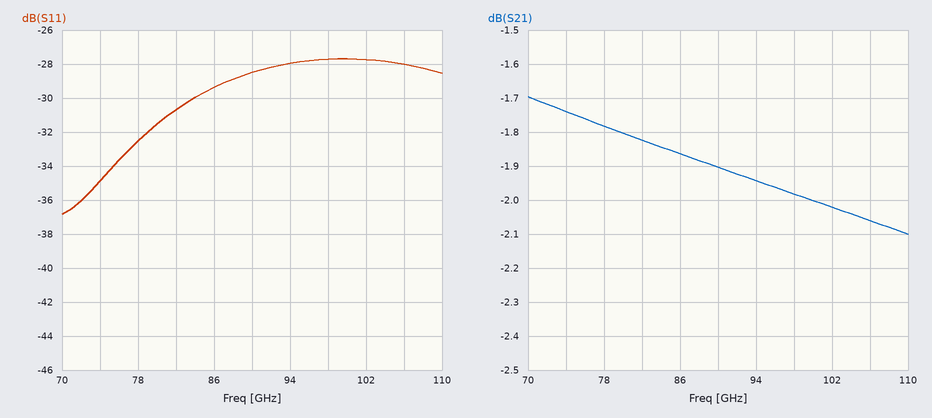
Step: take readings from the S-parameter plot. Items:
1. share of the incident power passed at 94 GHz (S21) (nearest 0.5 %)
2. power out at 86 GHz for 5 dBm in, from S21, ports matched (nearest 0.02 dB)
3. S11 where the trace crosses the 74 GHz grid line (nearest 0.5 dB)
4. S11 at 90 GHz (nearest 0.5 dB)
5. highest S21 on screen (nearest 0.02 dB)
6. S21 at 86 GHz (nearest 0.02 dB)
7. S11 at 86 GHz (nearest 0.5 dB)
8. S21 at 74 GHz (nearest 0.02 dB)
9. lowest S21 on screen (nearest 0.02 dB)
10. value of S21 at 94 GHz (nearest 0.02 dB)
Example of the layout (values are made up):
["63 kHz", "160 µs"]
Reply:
["64.0 %", "3.14 dBm", "-35.0 dB", "-28.5 dB", "-1.70 dB", "-1.86 dB", "-29.5 dB", "-1.74 dB", "-2.10 dB", "-1.94 dB"]
